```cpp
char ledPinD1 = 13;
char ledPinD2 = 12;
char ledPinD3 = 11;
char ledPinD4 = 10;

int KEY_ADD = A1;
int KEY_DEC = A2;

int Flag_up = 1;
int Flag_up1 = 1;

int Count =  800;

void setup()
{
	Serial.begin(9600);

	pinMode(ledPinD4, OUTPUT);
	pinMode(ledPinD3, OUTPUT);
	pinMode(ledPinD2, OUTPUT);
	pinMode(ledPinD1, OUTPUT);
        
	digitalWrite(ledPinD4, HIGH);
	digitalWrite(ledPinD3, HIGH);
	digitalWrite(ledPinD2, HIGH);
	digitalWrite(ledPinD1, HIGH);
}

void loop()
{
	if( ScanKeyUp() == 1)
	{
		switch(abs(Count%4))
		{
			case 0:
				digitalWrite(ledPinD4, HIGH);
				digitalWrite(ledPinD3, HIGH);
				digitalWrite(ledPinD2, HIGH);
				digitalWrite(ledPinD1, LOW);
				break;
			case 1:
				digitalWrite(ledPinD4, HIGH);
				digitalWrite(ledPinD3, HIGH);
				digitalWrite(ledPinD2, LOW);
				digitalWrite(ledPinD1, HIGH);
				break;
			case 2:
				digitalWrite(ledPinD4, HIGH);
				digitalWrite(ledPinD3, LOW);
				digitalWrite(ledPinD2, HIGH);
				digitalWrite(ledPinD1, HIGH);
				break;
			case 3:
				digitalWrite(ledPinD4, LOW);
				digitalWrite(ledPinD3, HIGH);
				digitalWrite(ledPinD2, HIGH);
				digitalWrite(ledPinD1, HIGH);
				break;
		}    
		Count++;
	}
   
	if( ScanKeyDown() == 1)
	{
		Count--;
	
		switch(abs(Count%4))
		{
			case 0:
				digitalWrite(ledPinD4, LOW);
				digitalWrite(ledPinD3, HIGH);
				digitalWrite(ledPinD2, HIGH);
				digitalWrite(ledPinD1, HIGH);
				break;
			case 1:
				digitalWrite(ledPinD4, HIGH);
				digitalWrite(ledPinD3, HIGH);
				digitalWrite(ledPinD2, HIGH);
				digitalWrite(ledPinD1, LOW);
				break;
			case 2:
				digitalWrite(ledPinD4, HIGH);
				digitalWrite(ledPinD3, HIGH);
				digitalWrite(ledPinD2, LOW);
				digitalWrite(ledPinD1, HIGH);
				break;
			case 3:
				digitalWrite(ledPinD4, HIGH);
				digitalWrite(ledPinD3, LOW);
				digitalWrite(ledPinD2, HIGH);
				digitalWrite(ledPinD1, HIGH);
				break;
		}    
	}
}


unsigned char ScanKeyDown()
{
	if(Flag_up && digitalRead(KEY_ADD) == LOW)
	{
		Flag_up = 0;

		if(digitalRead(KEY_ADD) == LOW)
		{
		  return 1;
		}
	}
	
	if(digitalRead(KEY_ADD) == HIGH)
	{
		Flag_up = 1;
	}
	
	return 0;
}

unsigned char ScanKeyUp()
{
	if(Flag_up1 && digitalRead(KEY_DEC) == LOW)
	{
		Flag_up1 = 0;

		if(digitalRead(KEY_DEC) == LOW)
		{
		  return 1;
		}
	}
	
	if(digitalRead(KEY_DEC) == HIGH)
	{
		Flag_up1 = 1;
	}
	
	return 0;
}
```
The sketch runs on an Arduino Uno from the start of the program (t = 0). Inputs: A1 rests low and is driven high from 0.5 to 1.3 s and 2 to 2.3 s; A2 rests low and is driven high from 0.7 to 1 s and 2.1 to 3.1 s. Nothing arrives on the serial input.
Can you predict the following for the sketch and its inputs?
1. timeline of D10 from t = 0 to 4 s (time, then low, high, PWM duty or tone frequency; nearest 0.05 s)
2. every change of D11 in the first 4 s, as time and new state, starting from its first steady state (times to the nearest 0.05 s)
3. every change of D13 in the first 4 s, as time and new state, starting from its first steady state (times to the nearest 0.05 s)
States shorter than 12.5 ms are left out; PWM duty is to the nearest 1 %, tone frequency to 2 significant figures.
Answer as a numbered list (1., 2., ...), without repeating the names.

1. 0 s low; 1 s high; 1.3 s low; 2.3 s high; 3.1 s low
2. 0 s high; 2.3 s low; 3.1 s high
3. 0 s high; 1 s low; 1.3 s high
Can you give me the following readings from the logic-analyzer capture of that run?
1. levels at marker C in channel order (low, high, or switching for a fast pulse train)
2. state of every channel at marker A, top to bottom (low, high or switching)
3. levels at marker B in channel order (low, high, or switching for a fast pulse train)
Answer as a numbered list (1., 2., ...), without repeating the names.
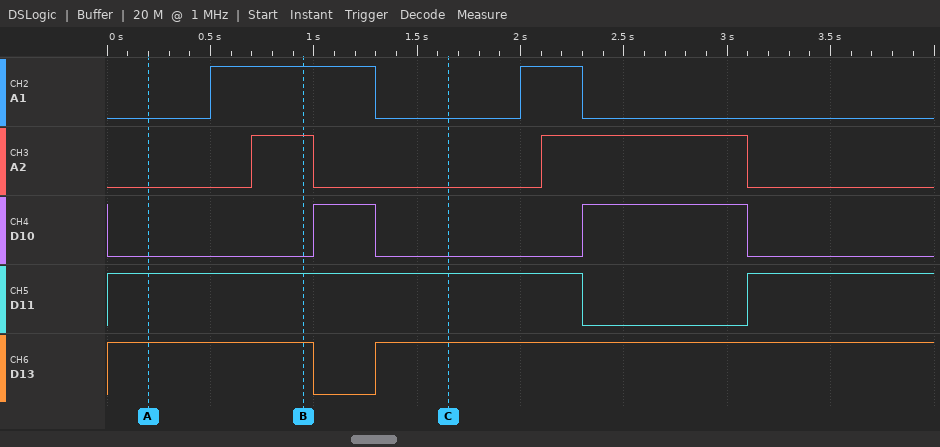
1. A1 low, A2 low, D10 low, D11 high, D13 high
2. A1 low, A2 low, D10 low, D11 high, D13 high
3. A1 high, A2 high, D10 low, D11 high, D13 high
